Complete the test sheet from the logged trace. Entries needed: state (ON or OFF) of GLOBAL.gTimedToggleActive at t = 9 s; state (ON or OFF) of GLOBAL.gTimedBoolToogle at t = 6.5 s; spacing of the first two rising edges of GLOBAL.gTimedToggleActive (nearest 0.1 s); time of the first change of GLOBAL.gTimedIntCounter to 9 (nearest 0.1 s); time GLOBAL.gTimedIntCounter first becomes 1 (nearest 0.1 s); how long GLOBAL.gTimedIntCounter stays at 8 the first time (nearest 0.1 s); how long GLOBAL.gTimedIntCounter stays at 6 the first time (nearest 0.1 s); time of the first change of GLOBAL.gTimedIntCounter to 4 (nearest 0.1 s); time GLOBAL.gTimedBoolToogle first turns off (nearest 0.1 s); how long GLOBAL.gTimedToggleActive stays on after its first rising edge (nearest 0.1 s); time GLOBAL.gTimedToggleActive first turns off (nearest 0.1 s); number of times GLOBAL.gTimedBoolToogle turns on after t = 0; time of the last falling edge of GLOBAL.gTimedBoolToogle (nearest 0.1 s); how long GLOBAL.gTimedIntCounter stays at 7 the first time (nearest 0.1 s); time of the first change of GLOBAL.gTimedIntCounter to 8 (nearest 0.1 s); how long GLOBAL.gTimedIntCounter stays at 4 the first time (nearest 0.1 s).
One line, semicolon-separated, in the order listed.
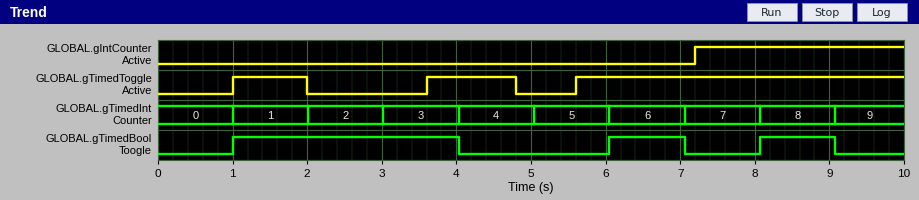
ON; ON; 2.6 s; 9.1 s; 1.0 s; 1.0 s; 1.0 s; 4.0 s; 4.0 s; 1.0 s; 2.0 s; 3; 9.1 s; 1.0 s; 8.1 s; 1.0 s
